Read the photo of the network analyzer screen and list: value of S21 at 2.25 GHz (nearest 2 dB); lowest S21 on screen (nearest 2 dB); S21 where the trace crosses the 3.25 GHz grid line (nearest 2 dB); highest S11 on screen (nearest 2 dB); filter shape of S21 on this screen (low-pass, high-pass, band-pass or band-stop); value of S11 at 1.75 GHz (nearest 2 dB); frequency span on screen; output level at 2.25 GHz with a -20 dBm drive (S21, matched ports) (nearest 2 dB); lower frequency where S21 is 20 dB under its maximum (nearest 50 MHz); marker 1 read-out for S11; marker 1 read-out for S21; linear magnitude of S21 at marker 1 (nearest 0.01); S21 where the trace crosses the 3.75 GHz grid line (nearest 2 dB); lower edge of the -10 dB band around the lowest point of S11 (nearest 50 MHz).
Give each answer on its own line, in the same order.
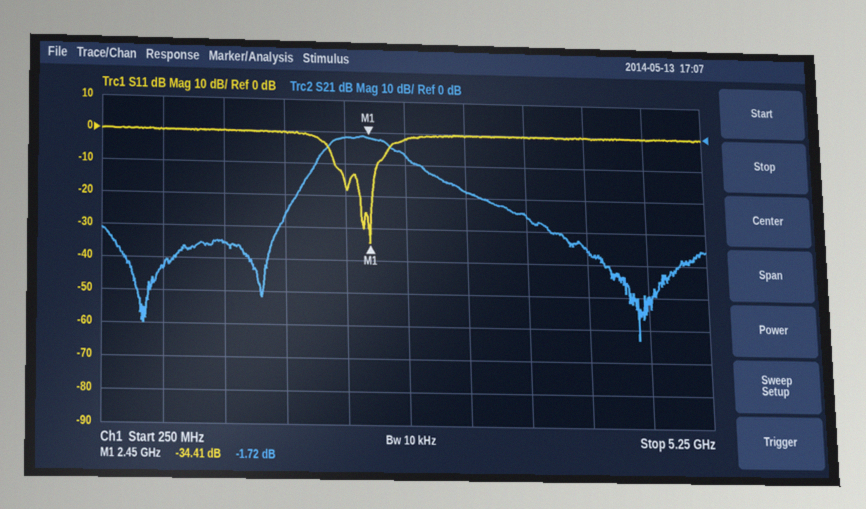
-2 dB
-64 dB
-18 dB
0 dB
band-pass
0 dB
5 GHz
-22 dBm
1.85 GHz
-34.41 dB
-1.72 dB
0.82
-26 dB
2.15 GHz
